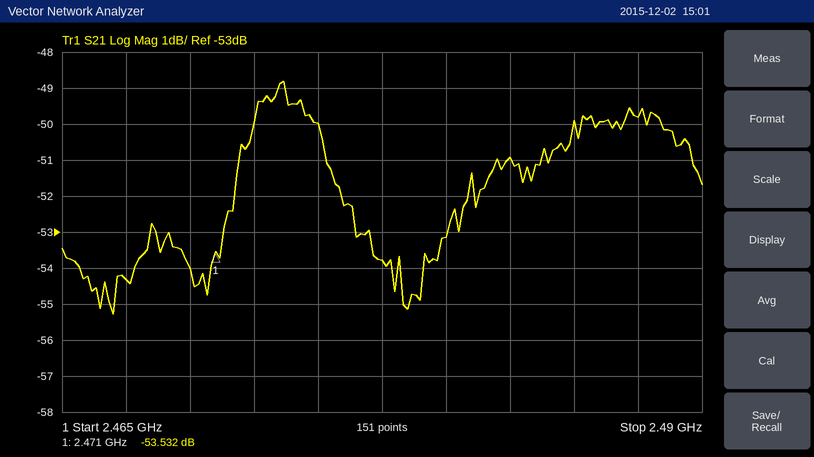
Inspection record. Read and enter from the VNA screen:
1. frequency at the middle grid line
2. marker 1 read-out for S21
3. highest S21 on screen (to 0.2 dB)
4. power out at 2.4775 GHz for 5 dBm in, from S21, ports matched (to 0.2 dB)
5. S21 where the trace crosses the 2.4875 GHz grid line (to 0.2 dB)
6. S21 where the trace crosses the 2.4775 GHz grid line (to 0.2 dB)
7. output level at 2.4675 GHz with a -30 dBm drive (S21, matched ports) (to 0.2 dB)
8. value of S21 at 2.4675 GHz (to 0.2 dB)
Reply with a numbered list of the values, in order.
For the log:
1. 2.4775 GHz
2. -53.532 dB
3. -48.8 dB
4. -48.8 dBm
5. -49.8 dB
6. -53.8 dB
7. -84.4 dBm
8. -54.4 dB
